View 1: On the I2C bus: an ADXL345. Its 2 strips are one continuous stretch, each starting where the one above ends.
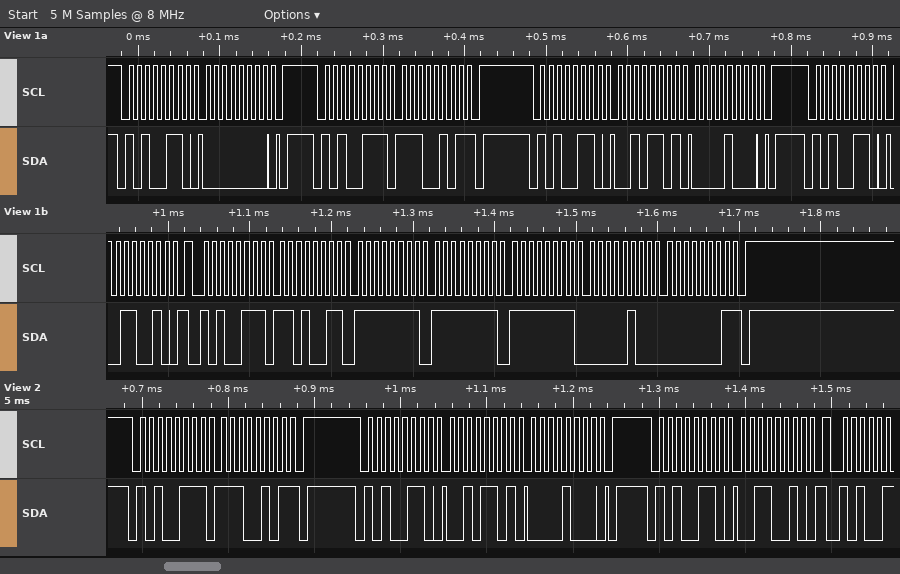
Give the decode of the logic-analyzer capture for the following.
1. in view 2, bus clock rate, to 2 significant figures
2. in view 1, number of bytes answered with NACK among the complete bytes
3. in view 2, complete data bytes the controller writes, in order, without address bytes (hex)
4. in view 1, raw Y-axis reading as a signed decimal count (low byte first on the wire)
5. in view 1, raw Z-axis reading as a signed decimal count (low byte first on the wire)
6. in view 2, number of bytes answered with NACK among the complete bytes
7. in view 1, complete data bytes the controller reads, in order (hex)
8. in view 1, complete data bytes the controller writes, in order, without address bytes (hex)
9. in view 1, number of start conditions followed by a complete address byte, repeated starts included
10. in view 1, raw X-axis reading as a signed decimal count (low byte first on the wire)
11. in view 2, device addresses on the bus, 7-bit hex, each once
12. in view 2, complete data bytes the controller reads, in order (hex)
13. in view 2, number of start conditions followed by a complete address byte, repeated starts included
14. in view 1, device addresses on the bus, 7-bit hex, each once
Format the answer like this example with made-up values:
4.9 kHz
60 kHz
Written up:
100 kHz
2
2D 08 32
-1
260
1
E5 D3 FF FF FF 04 01
00 2D 08 32
5
-45
0x53
E5
3
0x53
